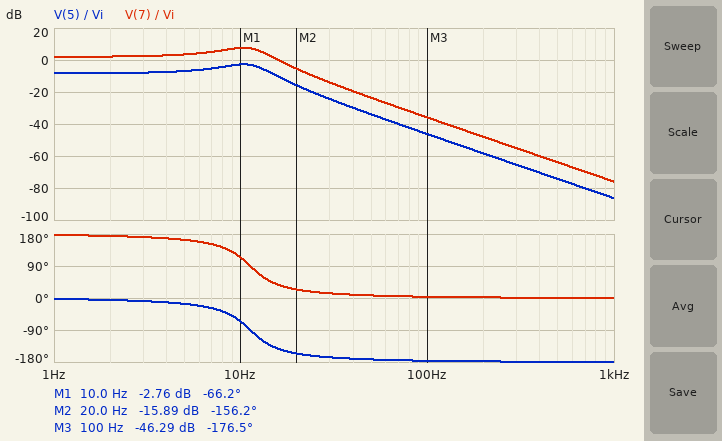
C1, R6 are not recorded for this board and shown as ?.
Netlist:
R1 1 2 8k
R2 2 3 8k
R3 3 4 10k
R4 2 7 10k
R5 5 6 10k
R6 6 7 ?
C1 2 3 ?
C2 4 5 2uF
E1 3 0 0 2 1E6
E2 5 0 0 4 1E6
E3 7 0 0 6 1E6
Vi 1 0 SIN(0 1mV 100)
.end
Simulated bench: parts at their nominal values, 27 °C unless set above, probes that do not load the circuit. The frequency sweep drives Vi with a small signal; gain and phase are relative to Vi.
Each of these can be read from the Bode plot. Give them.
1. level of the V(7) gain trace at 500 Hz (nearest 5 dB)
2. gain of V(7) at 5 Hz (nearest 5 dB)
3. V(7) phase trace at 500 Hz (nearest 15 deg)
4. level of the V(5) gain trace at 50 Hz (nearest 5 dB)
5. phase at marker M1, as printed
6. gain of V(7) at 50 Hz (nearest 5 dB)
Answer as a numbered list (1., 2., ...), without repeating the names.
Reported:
1. -65 dB
2. 5 dB
3. 0 deg
4. -35 dB
5. -66.2 deg
6. -25 dB
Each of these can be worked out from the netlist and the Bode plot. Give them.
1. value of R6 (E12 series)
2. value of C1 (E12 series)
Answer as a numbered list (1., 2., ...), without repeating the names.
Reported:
1. 33 kΩ
2. 3.3 µF
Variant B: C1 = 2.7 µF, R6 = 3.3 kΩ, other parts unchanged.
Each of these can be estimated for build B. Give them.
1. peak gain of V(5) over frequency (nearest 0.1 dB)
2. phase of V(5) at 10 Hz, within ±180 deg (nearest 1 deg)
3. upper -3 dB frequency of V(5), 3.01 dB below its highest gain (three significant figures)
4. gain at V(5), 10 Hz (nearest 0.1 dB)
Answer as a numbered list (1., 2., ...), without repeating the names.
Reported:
1. 11.6 dB
2. -139 deg
3. 2.78 Hz
4. -5.6 dB
